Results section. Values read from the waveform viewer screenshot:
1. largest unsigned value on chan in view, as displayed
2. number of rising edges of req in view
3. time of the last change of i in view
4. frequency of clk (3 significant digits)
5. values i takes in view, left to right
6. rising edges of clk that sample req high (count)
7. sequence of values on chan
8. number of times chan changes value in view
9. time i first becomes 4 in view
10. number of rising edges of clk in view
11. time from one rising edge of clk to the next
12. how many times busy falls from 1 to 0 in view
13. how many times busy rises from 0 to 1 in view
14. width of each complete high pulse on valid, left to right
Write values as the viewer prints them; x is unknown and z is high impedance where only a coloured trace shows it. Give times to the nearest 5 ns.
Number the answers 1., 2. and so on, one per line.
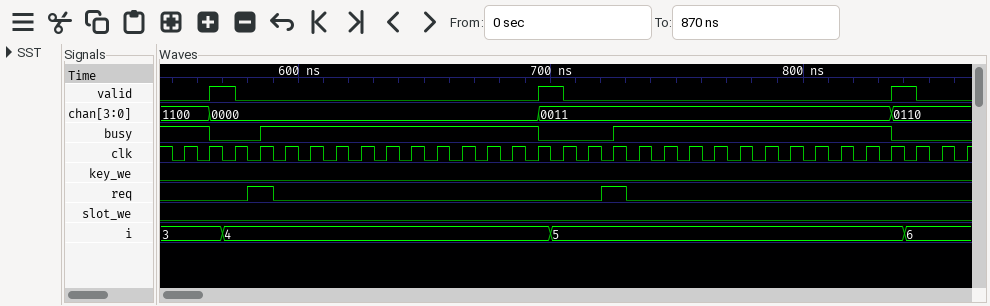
1. 1100
2. 2
3. 840 ns
4. 100 MHz
5. 3, 4, 5, 6
6. 2
7. 1100, 0000, 0011, 0110
8. 3
9. 570 ns
10. 32
11. 10 ns
12. 3
13. 2
14. 10 ns, 10 ns, 10 ns
